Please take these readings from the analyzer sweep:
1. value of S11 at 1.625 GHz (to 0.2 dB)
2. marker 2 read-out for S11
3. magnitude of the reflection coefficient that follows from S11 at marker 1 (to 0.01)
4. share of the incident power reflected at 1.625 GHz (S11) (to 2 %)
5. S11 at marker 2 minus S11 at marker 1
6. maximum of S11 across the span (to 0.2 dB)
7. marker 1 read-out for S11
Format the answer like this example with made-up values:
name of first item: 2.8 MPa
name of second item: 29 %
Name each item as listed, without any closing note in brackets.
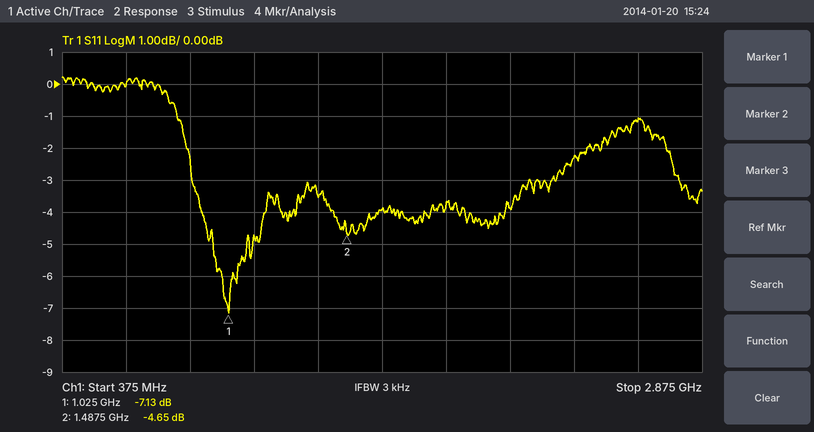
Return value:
value of S11 at 1.625 GHz: -4.0 dB
marker 2 read-out for S11: -4.65 dB
magnitude of the reflection coefficient that follows from S11 at marker 1: 0.44
share of the incident power reflected at 1.625 GHz (S11): 40 %
S11 at marker 2 minus S11 at marker 1: 2.48 dB
maximum of S11 across the span: 0.2 dB
marker 1 read-out for S11: -7.13 dB
